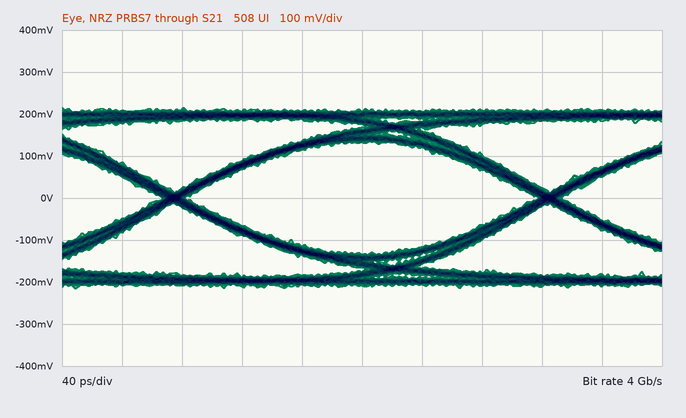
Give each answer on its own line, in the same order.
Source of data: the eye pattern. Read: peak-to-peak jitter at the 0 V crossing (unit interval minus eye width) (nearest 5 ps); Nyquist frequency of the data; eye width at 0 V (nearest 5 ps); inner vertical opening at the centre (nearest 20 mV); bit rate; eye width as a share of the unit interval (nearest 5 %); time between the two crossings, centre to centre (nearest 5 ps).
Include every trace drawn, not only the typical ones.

15 ps
2 GHz
235 ps
260 mV
4 Gb/s
95 %
250 ps
